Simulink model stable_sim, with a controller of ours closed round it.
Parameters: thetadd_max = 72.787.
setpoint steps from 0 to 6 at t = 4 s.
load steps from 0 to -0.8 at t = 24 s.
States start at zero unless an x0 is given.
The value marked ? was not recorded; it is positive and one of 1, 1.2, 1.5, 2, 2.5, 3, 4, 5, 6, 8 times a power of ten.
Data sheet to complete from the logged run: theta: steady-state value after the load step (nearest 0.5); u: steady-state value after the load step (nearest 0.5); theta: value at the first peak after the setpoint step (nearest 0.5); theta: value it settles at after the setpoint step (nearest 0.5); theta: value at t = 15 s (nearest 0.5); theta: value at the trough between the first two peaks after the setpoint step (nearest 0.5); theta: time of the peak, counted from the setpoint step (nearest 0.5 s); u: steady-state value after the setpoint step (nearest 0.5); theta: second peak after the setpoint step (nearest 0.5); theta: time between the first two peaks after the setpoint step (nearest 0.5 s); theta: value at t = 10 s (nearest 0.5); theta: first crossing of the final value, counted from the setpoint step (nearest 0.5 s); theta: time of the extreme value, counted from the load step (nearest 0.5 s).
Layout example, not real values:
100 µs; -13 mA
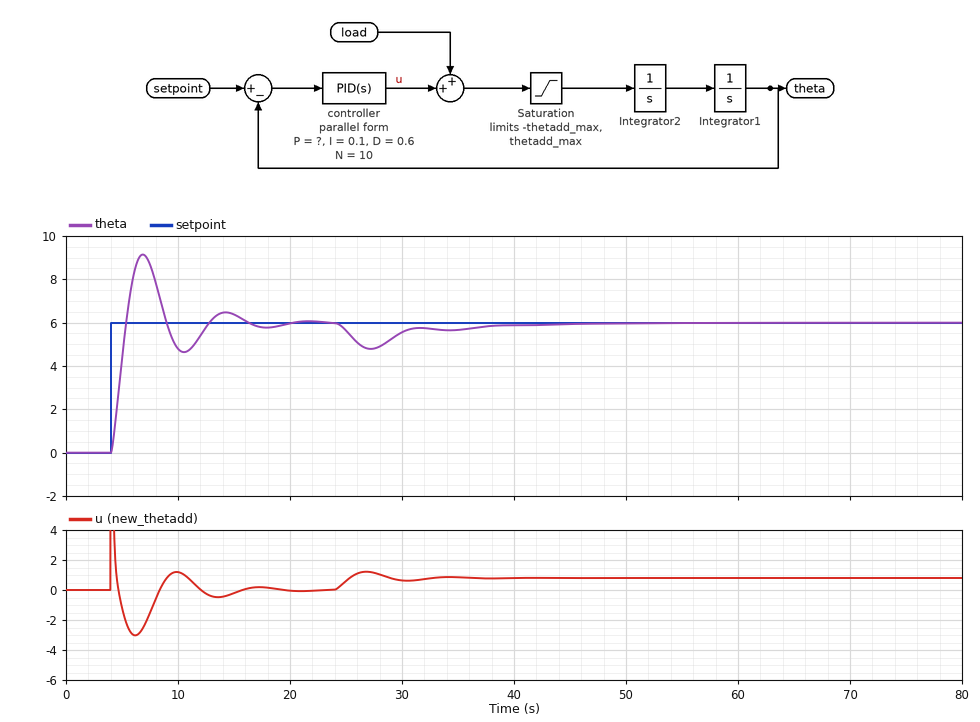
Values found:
6.0; 1.0; 9.0; 6.0; 6.5; 4.5; 3.0 s; 0.0; 6.5; 7.5 s; 5.0; 1.5 s; 3.0 s
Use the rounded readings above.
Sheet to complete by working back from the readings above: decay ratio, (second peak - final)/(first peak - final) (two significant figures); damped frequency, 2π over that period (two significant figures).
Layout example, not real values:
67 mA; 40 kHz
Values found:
0.17; 0.84 rad/s
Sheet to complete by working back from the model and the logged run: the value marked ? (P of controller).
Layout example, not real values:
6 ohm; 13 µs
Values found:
0.8
